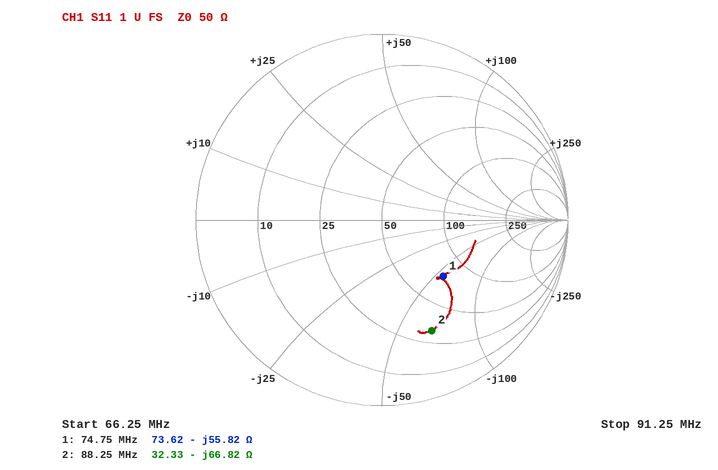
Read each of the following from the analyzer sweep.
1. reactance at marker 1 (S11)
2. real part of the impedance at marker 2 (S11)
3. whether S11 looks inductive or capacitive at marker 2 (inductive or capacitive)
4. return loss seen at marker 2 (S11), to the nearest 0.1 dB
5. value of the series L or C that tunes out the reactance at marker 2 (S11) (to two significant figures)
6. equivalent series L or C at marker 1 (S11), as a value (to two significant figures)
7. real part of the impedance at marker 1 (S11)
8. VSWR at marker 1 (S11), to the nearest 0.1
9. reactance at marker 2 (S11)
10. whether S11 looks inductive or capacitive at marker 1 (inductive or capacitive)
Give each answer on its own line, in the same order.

-55.82 Ω
32.33 Ω
capacitive
3.7 dB
120 nH
38 pF
73.62 Ω
2.6
-66.82 Ω
capacitive
